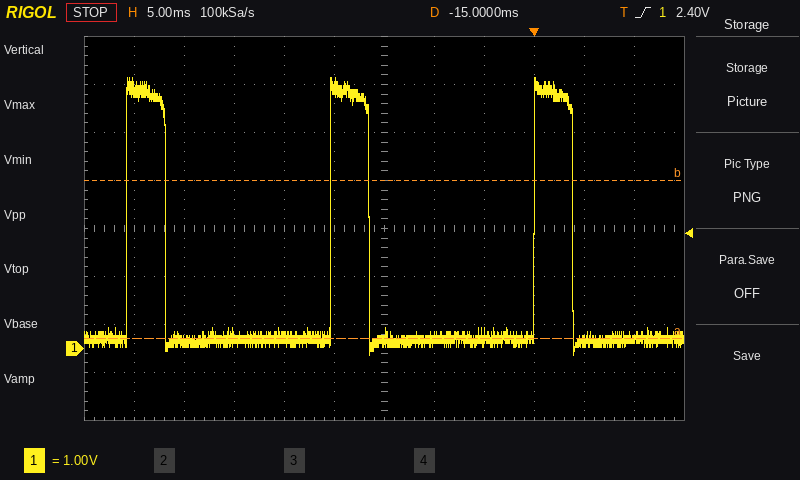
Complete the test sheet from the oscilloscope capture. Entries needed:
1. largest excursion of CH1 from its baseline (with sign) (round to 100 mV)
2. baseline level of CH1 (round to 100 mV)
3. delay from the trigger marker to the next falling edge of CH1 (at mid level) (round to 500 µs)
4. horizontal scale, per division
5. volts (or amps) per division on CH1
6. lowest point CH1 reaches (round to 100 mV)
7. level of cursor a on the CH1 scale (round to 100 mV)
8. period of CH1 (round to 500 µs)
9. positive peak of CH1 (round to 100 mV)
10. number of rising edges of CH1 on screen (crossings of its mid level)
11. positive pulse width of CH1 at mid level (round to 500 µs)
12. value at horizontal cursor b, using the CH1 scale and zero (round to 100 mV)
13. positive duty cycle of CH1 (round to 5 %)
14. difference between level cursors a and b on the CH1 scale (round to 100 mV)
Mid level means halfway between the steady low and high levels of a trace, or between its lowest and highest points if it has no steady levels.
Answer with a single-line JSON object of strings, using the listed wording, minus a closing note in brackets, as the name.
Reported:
{"largest excursion of CH1 from its baseline (with sign)": "+5.4 V", "baseline level of CH1": "200 mV", "delay from the trigger marker to the next falling edge of CH1 (at mid level)": "4.0 ms", "horizontal scale, per division": "5 ms", "volts (or amps) per division on CH1": "1 V", "lowest point CH1 reaches": "-100 mV", "level of cursor a on the CH1 scale": "200 mV", "period of CH1": "20.5 ms", "positive peak of CH1": "5.6 V", "number of rising edges of CH1 on screen": "3", "positive pulse width of CH1 at mid level": "4.0 ms", "value at horizontal cursor b, using the CH1 scale and zero": "3.5 V", "positive duty cycle of CH1": "20 %", "difference between level cursors a and b on the CH1 scale": "3.3 V"}
